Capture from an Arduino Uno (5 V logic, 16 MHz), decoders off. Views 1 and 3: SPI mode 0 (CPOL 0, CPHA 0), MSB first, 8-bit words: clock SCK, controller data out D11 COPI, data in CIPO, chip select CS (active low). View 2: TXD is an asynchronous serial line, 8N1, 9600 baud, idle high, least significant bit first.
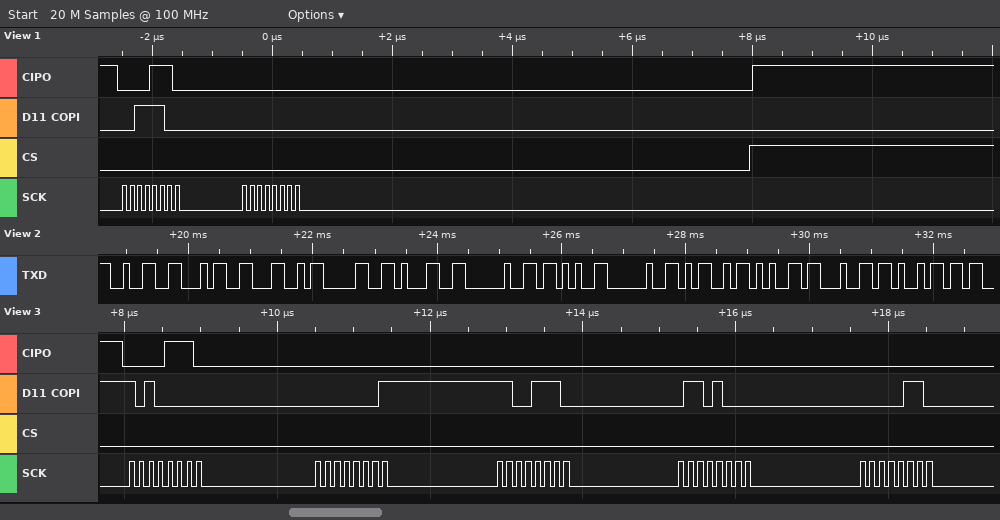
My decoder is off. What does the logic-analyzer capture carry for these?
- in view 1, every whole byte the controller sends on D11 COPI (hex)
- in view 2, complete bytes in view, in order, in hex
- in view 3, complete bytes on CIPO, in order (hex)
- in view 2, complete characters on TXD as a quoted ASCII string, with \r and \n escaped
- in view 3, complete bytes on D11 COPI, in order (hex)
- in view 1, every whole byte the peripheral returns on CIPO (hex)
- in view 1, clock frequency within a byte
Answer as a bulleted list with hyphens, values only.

- 3C 00
- 0x32 0x34 0x4C 0x30 0x31 0x20 0x2B 0x20 0x4D 0x65 0x64 0x69
- 0E 00 00 00 00
- "24L01 + Medi"
- A0 01 CE 68 06
- 0E 00
- 8 MHz
